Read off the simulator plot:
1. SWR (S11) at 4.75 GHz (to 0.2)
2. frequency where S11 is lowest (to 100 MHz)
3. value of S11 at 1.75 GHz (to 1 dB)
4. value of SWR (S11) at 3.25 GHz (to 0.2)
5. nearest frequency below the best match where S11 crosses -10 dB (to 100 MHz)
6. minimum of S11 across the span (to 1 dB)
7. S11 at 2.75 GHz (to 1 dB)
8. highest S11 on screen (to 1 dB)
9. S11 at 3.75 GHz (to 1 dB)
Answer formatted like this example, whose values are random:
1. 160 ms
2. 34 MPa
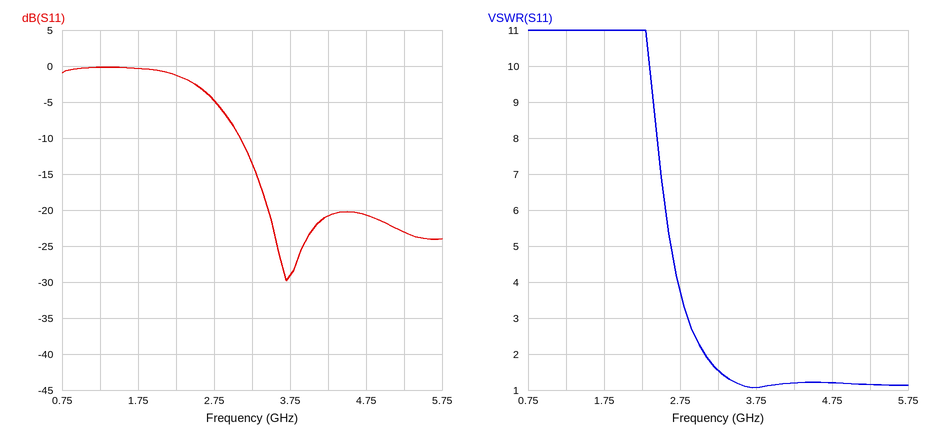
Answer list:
1. 1.2
2. 3.7 GHz
3. 0 dB
4. 1.6
5. 3.1 GHz
6. -30 dB
7. -5 dB
8. 0 dB
9. -29 dB
